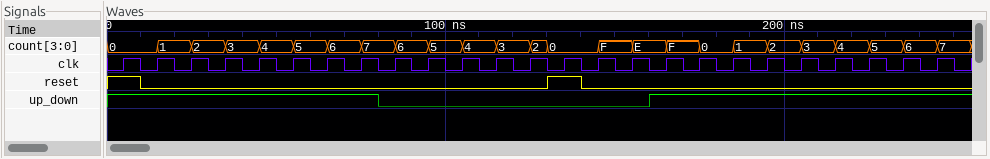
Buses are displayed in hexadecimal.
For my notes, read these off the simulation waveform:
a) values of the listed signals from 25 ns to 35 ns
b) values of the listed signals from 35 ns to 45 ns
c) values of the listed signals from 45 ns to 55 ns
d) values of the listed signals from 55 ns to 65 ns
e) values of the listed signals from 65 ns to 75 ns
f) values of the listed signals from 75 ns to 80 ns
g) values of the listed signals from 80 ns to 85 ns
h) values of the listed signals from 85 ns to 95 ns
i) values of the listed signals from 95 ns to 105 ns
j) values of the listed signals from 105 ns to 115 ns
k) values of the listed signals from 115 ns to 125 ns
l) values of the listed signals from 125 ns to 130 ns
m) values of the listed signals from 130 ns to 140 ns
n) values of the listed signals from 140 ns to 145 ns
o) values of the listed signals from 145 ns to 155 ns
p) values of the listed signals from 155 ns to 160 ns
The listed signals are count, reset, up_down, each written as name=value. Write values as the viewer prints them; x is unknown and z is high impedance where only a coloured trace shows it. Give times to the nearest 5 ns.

count=2, reset=0, up_down=1
count=3, reset=0, up_down=1
count=4, reset=0, up_down=1
count=5, reset=0, up_down=1
count=6, reset=0, up_down=1
count=7, reset=0, up_down=1
count=7, reset=0, up_down=0
count=6, reset=0, up_down=0
count=5, reset=0, up_down=0
count=4, reset=0, up_down=0
count=3, reset=0, up_down=0
count=2, reset=0, up_down=0
count=0, reset=1, up_down=0
count=0, reset=0, up_down=0
count=F, reset=0, up_down=0
count=E, reset=0, up_down=0
